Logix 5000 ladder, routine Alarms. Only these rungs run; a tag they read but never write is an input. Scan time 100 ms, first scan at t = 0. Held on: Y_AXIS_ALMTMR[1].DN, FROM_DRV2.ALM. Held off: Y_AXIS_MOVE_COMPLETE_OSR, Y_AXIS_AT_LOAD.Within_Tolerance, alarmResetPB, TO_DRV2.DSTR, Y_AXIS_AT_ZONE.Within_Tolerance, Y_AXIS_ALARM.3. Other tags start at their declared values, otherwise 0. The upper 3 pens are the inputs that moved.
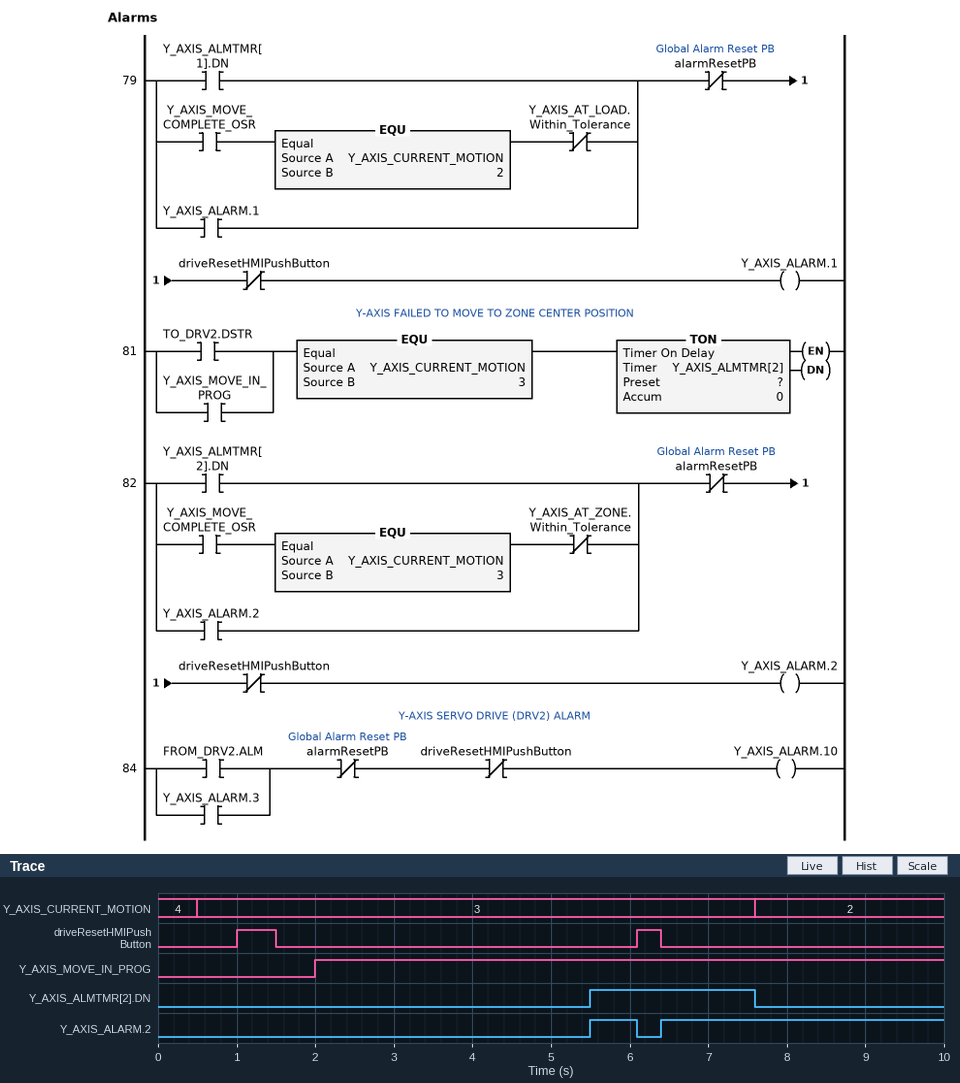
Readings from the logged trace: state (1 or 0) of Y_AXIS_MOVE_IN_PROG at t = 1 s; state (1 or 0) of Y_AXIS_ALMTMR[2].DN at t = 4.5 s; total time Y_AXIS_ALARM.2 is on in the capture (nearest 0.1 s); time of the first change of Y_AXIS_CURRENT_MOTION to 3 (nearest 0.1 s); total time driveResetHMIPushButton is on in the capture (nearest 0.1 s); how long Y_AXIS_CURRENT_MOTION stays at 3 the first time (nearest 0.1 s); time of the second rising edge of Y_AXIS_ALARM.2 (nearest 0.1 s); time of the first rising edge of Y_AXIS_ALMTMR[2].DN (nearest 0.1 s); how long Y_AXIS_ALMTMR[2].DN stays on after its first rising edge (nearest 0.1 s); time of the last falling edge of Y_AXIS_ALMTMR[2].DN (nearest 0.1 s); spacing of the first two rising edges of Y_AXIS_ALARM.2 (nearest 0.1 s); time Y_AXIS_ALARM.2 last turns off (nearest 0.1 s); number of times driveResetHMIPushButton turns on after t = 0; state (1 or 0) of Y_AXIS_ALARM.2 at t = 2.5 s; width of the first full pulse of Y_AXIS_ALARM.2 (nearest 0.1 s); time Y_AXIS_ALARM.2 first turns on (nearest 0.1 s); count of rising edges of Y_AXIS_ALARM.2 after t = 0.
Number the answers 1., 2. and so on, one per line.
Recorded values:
1. 0
2. 0
3. 4.2 s
4. 0.5 s
5. 0.8 s
6. 7.1 s
7. 6.4 s
8. 5.5 s
9. 2.1 s
10. 7.6 s
11. 0.9 s
12. 6.1 s
13. 2
14. 0
15. 0.6 s
16. 5.5 s
17. 2
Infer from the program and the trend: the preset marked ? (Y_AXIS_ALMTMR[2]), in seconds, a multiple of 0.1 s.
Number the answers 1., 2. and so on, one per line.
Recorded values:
1. 3.5 s
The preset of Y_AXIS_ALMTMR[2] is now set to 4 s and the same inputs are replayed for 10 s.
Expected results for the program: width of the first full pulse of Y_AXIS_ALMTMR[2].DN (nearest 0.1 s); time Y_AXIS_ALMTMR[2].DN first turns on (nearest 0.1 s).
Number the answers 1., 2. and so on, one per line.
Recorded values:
1. 1.6 s
2. 6.0 s
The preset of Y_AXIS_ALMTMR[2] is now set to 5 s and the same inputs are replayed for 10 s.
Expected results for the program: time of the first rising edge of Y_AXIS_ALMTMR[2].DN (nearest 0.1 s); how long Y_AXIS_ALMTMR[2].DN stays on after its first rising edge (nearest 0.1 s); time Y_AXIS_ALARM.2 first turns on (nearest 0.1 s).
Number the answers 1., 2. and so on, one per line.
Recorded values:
1. 7.0 s
2. 0.6 s
3. 7.0 s
